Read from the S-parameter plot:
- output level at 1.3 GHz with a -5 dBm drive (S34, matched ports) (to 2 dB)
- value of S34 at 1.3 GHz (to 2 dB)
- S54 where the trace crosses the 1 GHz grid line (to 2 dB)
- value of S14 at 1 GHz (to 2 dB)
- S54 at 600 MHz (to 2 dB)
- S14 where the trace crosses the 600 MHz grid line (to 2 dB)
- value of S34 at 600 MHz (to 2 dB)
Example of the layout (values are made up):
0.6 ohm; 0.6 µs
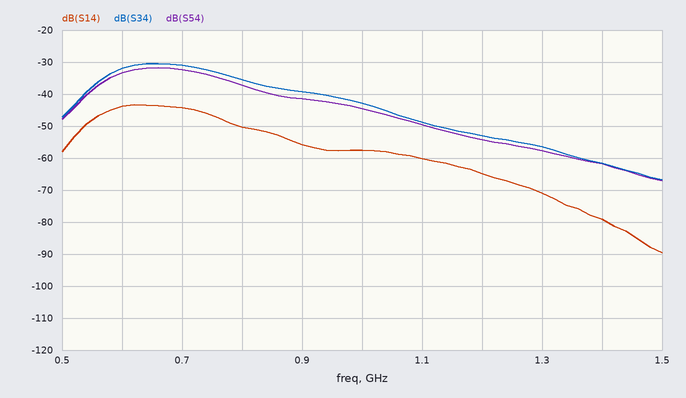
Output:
-62 dBm; -56 dB; -44 dB; -58 dB; -34 dB; -44 dB; -32 dB
